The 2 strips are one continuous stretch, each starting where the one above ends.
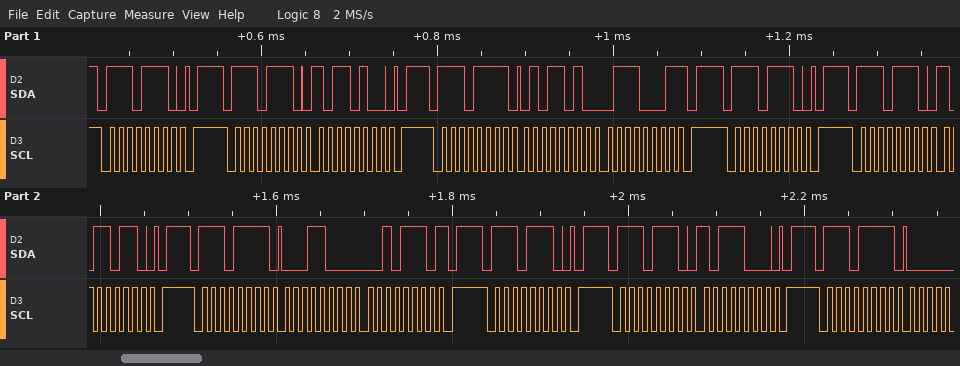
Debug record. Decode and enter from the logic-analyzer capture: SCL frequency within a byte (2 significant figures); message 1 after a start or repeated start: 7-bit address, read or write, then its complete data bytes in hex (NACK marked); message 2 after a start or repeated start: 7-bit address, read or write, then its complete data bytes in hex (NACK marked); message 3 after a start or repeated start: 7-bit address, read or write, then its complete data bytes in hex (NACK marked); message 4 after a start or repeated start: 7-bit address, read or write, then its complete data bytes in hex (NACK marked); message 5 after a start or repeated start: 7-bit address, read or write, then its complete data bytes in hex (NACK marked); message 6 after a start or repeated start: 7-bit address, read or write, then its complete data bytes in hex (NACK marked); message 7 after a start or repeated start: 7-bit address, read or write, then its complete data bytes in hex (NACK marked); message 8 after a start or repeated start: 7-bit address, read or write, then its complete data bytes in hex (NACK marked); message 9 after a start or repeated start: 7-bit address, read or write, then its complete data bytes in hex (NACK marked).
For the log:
100 kHz
0x77 write
0x77 write: B4
0x77 read: 5A 71 NACK
0x77 write
0x77 write: B6
0x77 read: 18 2E NACK
0x77 write
0x77 write: B8
0x77 read
